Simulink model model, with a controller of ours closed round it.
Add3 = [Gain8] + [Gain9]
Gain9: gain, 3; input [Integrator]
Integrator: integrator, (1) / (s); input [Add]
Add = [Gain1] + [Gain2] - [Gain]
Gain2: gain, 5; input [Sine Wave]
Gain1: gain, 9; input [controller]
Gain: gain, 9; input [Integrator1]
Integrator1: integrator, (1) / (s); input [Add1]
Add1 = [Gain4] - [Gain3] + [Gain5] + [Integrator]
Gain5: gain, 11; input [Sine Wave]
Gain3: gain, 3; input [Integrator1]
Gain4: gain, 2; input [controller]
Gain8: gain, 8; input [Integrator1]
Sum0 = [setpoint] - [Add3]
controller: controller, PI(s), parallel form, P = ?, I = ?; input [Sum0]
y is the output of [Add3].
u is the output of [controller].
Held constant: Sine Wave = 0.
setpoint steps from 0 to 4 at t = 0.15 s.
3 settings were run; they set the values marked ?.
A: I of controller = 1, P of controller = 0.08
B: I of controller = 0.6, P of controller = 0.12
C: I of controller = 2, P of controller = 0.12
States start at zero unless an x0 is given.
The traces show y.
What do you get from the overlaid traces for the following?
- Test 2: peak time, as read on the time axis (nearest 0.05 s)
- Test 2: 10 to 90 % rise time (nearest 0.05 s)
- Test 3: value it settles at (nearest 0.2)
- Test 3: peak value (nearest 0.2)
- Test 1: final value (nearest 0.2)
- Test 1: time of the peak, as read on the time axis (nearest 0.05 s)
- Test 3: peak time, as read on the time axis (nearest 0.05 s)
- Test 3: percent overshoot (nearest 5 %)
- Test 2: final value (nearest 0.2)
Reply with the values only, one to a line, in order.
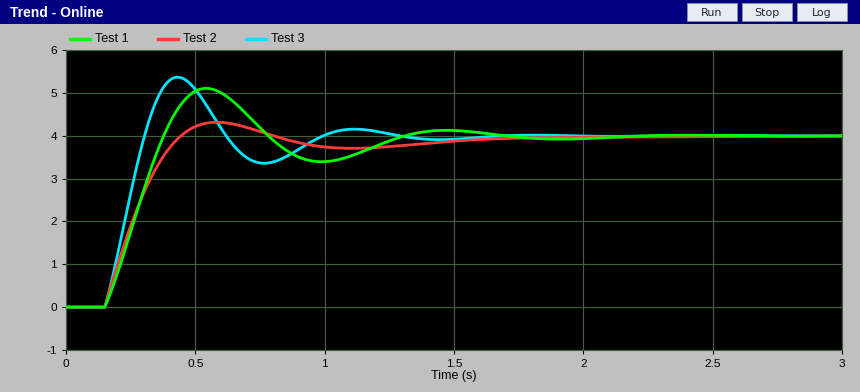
0.60 s
0.20 s
4.0
5.4
4.0
0.55 s
0.45 s
35 %
4.0
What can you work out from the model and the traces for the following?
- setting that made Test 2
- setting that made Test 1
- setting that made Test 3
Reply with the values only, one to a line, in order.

B
A
C
